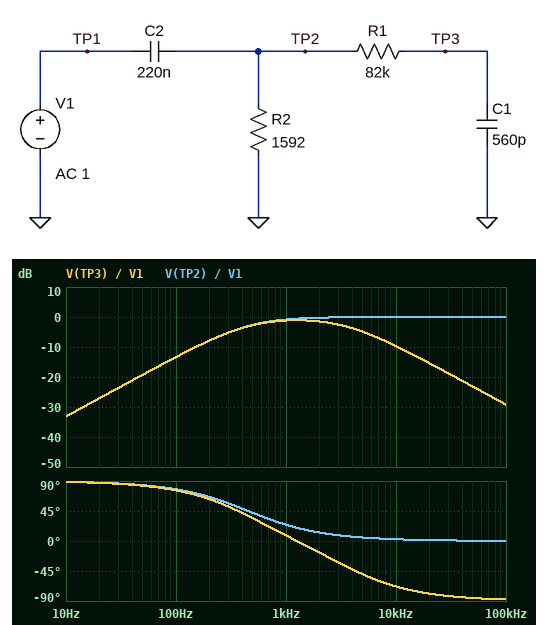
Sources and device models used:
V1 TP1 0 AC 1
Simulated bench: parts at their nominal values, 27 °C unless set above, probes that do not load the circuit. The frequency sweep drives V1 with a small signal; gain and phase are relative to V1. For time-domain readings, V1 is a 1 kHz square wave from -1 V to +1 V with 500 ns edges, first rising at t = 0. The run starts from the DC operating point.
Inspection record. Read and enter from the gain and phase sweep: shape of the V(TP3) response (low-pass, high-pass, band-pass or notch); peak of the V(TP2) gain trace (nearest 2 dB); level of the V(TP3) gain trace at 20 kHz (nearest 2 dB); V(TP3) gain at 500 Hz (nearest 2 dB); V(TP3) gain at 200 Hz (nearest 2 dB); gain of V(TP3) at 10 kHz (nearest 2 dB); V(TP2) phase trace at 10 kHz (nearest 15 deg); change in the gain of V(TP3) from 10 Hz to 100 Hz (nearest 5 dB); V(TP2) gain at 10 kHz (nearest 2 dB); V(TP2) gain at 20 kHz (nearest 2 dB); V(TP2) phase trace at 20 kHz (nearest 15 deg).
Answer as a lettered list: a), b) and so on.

a) band-pass
b) 0 dB
c) -16 dB
d) -2 dB
e) -8 dB
f) -10 dB
g) 0 deg
h) 20 dB
i) 0 dB
j) 0 dB
k) 0 deg
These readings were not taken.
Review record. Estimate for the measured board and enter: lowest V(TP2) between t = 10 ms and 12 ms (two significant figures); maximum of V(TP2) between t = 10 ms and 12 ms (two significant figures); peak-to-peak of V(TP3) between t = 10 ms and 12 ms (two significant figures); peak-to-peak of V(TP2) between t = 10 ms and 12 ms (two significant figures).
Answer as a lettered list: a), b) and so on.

a) -1.6 V
b) 1.6 V
c) 2.3 V
d) 3.2 V
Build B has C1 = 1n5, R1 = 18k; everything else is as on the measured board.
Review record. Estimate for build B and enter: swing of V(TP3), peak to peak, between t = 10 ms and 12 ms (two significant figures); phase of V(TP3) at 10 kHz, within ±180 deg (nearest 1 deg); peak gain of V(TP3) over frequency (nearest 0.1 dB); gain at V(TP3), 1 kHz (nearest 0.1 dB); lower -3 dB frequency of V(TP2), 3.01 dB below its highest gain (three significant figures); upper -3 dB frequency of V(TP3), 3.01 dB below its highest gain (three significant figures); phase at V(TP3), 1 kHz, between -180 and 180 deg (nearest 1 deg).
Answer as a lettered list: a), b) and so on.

a) 2.5 V
b) -57 deg
c) -0.7 dB
d) -1.0 dB
e) 458 Hz
f) 6.78 kHz
g) 15 deg
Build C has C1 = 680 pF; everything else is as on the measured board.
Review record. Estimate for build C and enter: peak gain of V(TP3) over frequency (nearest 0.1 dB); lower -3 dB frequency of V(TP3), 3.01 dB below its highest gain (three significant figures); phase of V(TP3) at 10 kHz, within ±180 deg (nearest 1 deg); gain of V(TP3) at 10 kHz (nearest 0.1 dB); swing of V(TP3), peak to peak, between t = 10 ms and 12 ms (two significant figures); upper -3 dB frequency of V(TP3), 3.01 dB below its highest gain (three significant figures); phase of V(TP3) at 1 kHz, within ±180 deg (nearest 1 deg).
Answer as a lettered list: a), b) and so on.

a) -1.3 dB
b) 353 Hz
c) -71 deg
d) -11.2 dB
e) 2.2 V
f) 3.67 kHz
g) 5 deg
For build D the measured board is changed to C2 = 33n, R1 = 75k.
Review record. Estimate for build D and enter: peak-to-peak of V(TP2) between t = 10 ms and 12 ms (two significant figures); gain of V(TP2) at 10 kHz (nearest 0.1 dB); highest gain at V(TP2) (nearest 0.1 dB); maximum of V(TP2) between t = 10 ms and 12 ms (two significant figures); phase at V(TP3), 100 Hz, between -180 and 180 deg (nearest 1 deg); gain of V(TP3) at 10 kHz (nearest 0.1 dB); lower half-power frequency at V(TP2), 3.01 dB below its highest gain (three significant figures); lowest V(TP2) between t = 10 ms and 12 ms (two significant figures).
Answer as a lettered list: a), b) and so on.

a) 4.0 V
b) -0.4 dB
c) 0 dB
d) 2.0 V
e) 87 deg
f) -9.4 dB
g) 3.09 kHz
h) -2.0 V
